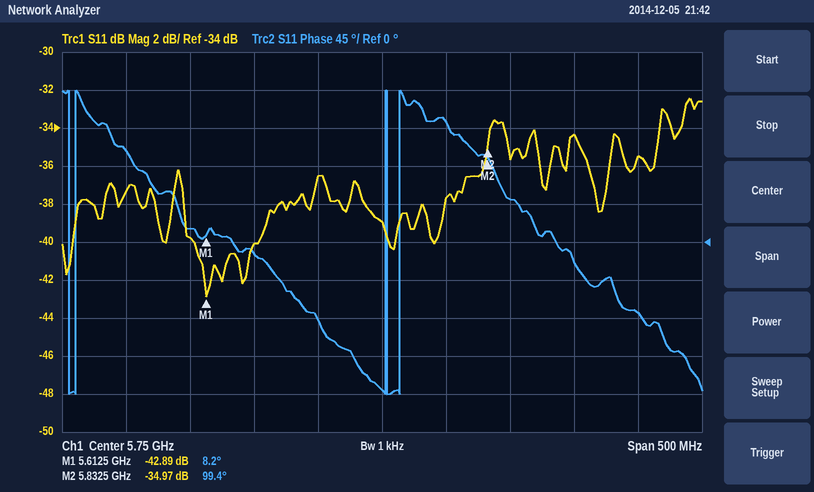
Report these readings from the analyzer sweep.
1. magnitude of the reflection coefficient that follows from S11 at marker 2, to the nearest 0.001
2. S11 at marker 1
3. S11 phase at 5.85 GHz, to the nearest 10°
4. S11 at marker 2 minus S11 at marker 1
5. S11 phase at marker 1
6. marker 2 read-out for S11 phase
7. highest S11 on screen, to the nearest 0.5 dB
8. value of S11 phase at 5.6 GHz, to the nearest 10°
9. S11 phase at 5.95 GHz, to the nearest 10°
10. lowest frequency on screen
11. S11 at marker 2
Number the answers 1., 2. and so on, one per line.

1. 0.018
2. -42.89 dB
3. 50°
4. 7.92 dB
5. 8.2°
6. 99.4°
7. -32.5 dB
8. 20°
9. -80°
10. 5.5 GHz
11. -34.97 dB
